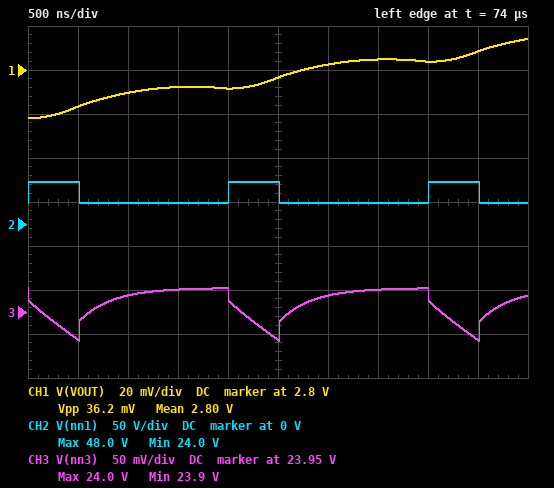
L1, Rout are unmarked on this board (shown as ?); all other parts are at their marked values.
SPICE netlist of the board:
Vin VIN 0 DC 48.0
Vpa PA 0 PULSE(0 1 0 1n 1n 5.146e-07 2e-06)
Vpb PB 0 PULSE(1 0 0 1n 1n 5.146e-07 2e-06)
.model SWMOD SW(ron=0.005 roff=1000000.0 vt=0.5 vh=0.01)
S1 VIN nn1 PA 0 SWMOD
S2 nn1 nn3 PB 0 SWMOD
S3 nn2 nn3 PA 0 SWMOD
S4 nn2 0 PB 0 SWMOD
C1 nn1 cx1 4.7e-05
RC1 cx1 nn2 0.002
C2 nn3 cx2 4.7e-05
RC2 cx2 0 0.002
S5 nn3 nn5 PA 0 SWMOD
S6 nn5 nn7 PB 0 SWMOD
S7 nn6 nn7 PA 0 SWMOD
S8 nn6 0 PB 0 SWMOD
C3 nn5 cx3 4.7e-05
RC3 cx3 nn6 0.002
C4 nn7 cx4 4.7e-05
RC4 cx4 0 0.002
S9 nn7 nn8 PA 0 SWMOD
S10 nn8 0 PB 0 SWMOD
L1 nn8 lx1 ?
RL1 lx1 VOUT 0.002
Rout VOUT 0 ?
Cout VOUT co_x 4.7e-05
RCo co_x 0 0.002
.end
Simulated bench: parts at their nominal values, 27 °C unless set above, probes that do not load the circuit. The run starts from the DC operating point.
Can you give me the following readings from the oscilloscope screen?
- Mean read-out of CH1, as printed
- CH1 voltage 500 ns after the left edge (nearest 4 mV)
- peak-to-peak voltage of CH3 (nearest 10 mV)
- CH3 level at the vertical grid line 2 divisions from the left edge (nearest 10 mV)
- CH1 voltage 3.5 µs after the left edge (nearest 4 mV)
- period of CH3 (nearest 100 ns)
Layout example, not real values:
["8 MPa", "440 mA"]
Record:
["2.80 V", "2.784 V", "60 mV", "23.97 V", "2.804 V", "2.0 µs"]
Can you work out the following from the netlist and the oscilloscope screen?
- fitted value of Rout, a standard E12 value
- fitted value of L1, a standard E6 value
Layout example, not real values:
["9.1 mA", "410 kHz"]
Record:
["0.15 Ω", "4.7 µH"]
